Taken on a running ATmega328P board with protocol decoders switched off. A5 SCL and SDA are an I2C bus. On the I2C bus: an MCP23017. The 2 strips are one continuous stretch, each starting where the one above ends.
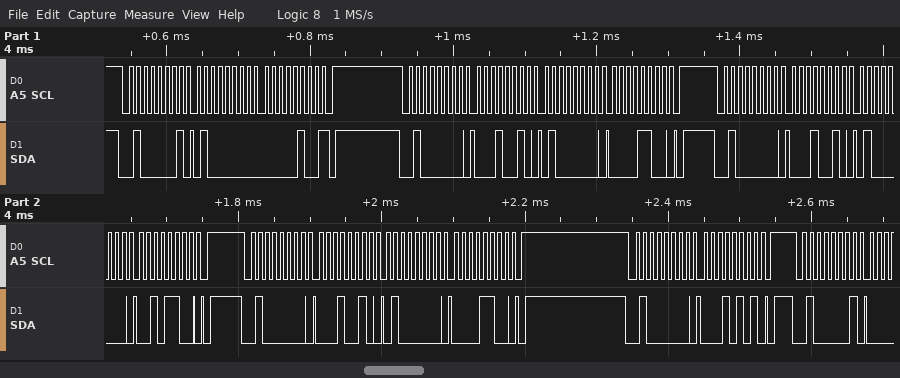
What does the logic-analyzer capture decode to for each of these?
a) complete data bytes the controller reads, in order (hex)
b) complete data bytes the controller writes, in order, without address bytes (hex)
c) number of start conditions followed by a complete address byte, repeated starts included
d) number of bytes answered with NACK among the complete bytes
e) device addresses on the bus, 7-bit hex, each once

40 04
12 40 0C 12 40 2C 12 40 0C 15
6
1
0x20
